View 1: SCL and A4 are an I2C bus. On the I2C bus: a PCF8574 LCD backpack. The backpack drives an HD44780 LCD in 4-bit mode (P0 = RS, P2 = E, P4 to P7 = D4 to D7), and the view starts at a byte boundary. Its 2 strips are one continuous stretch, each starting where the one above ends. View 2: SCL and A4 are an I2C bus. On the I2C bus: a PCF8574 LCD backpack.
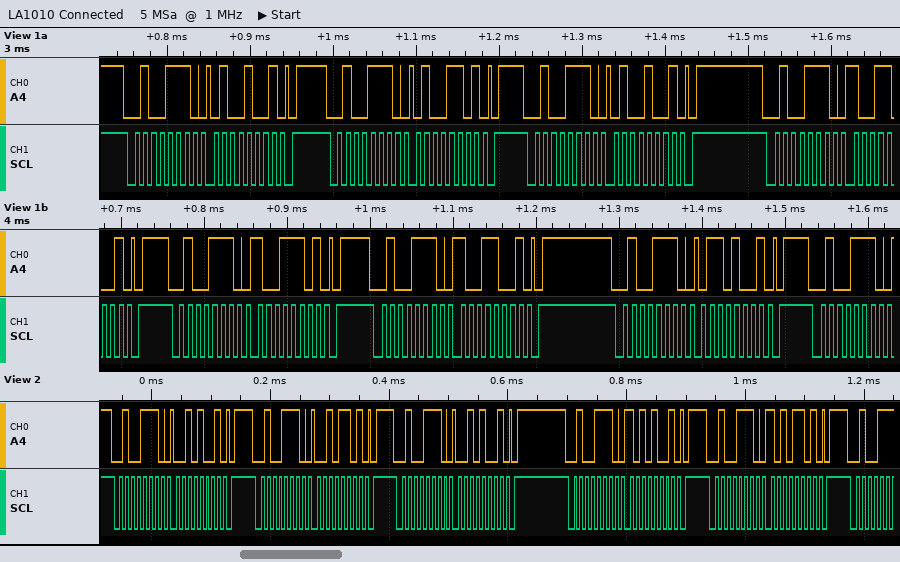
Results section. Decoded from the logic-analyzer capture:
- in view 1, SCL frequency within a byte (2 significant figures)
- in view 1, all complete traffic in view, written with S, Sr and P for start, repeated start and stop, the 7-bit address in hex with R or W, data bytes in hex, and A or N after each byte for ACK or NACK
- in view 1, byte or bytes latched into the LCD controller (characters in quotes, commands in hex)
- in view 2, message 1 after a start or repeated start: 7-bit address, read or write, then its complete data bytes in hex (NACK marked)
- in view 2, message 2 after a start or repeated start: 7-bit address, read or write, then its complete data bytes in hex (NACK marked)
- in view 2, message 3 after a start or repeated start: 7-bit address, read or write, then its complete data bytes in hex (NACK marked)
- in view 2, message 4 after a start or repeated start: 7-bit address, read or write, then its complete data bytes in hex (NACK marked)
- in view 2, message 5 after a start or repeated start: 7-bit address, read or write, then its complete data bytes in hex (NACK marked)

100 kHz
S 27W A 49 A P S 27W A 4D A P S 27W A 49 A P S 27W A 99 A P S 27W A 9D A P S 27W A 99 A P S 27W A 69 A P S 27W A
'I'
0x27 write: 29
0x27 write: 2D
0x27 write: 29
0x27 write: A9
0x27 write: AD
